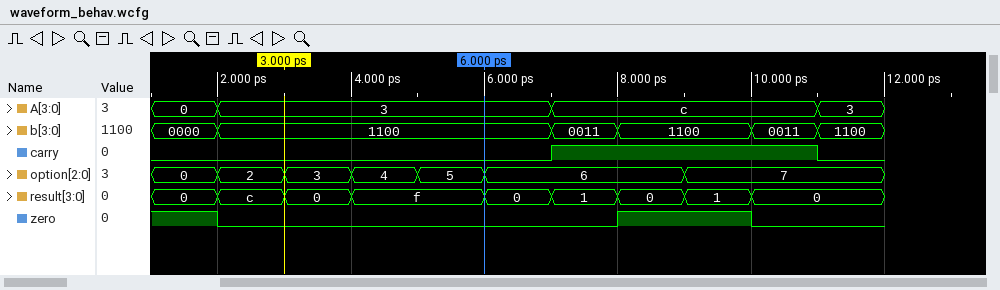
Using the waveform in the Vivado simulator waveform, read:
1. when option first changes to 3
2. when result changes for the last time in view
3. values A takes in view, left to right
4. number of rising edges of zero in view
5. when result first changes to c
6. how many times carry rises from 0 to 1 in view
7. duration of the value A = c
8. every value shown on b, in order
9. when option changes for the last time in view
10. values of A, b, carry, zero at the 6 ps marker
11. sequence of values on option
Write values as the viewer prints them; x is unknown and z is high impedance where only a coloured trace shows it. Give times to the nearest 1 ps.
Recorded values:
3 ps
10 ps
0, 3, c, 3
1
2 ps
1
4 ps
0000, 1100, 0011, 1100, 0011, 1100
9 ps
A=3, b=1100, carry=0, zero=0
0, 2, 3, 4, 5, 6, 7
